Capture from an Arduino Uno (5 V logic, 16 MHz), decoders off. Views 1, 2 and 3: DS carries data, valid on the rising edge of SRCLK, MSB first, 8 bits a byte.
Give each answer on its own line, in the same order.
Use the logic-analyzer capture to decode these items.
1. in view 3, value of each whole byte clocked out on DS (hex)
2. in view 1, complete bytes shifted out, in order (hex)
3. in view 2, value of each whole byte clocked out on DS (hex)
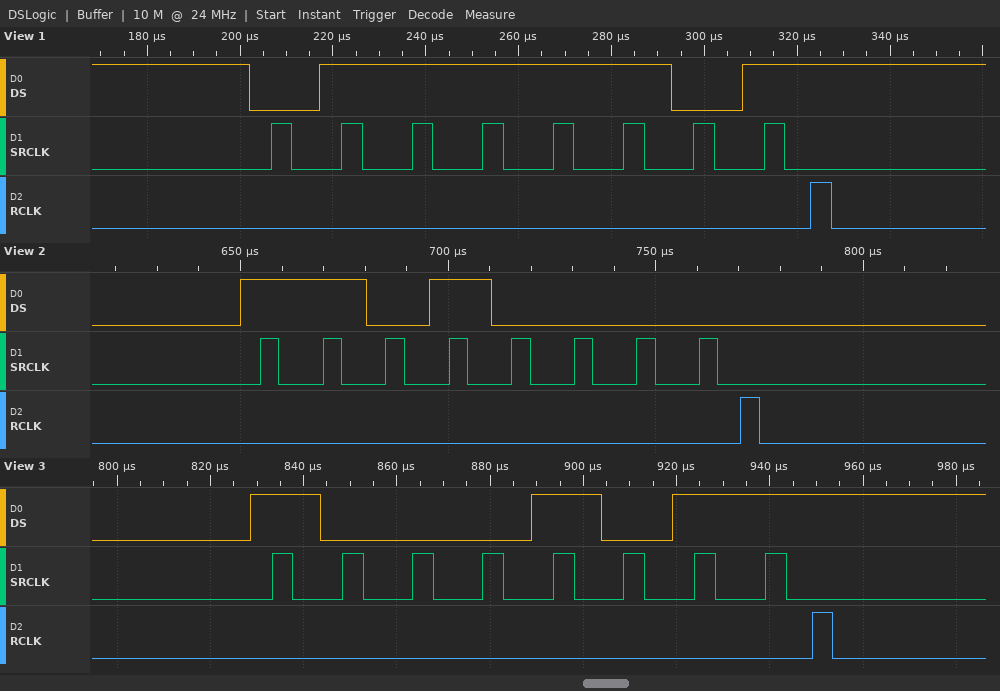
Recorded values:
8B
0x7D
D0
